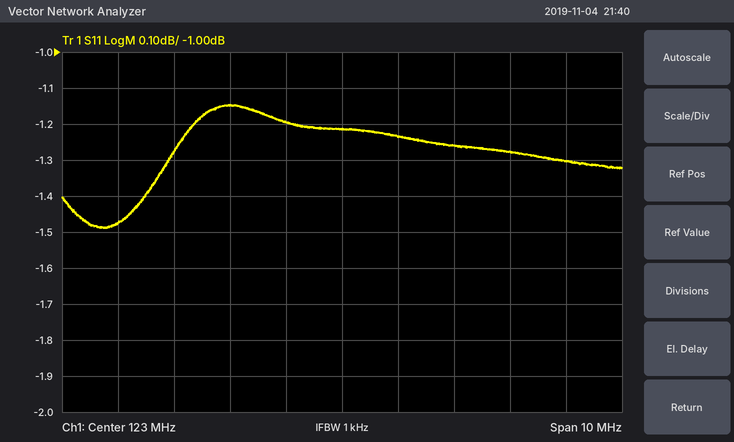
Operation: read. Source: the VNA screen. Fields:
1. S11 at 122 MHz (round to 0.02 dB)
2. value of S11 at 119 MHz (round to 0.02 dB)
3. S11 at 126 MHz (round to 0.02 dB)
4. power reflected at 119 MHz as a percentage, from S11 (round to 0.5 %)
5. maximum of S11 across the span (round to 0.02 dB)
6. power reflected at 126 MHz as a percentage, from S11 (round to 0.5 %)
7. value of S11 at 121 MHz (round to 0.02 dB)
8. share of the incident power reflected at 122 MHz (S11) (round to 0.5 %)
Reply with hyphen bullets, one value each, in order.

- -1.20 dB
- -1.48 dB
- -1.28 dB
- 71.0 %
- -1.14 dB
- 74.5 %
- -1.14 dB
- 76.0 %
